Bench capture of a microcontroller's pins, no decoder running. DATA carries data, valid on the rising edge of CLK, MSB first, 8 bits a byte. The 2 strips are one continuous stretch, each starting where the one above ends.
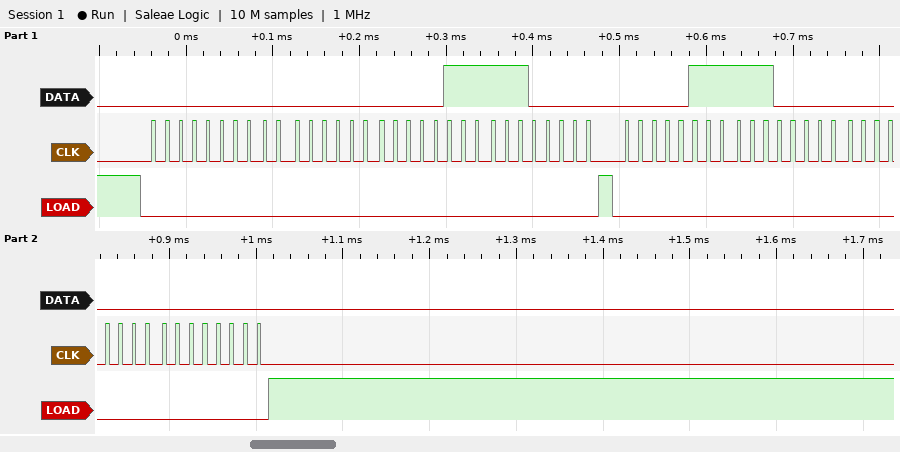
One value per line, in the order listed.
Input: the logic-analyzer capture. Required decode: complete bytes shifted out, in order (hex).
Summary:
00 00 07 E0 07 E0 00 00
